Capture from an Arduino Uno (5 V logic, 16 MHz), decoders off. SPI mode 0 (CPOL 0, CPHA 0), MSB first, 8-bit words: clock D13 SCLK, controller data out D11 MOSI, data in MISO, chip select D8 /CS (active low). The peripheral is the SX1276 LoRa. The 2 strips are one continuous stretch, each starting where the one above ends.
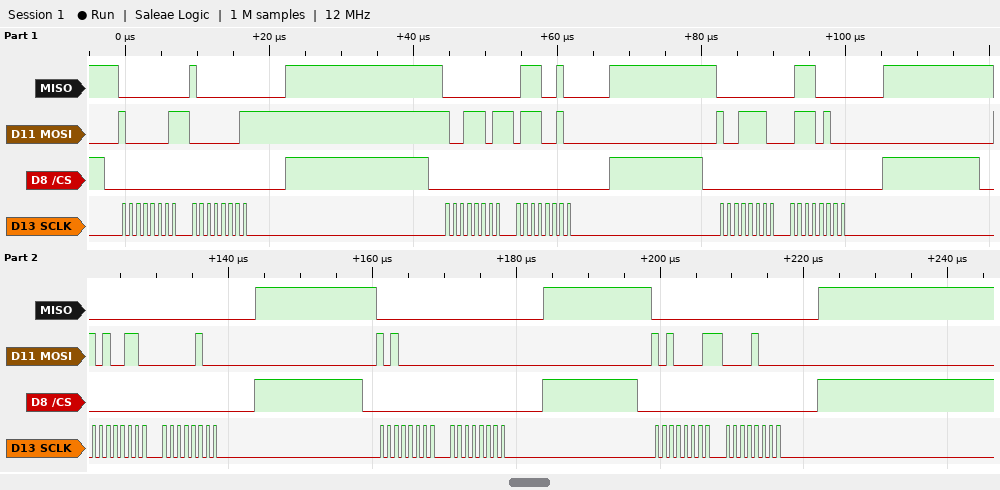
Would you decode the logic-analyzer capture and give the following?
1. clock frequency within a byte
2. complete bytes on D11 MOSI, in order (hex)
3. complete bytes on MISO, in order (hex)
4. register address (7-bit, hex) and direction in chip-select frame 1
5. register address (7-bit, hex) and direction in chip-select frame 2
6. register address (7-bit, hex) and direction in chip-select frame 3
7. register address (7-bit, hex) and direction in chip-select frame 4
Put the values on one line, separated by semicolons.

1 MHz; 81 01 9D 72 9E 74 A6 04 A0 00 A1 08; 00 80 00 72 00 70 00 00 00 00 00 00; 0x01 write; 0x1D write; 0x1E write; 0x26 write
